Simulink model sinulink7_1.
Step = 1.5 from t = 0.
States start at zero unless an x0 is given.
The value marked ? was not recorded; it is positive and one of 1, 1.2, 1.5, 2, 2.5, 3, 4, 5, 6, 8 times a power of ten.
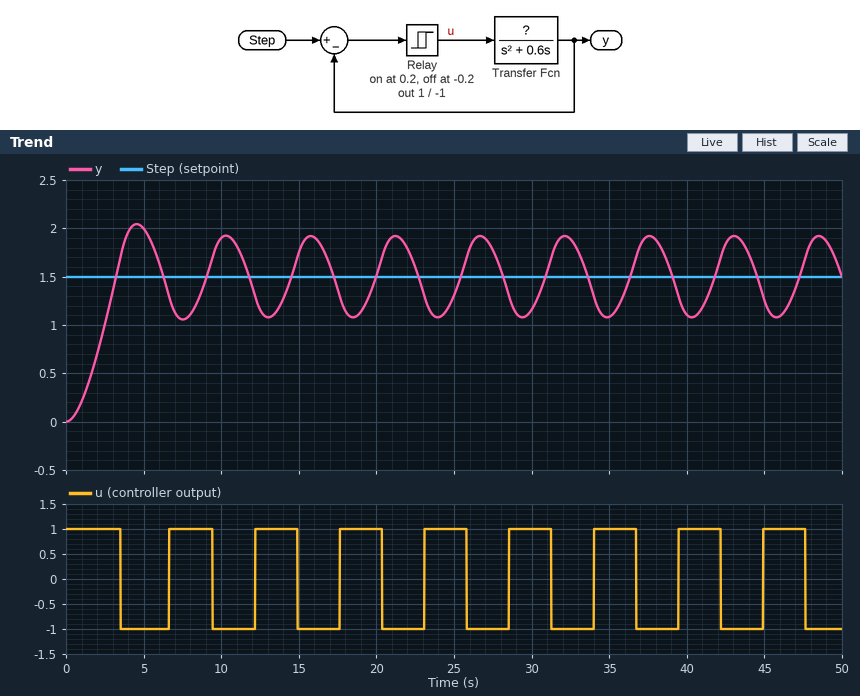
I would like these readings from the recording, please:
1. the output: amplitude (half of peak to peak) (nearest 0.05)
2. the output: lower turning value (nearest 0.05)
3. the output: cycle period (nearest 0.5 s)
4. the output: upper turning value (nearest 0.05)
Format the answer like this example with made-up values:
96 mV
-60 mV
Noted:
0.40
1.10
5.5 s
1.90
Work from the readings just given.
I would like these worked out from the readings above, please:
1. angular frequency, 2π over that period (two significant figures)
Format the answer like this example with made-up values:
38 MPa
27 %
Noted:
1.1 rad/s
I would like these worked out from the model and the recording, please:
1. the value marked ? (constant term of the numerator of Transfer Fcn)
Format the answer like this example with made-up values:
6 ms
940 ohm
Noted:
0.5
